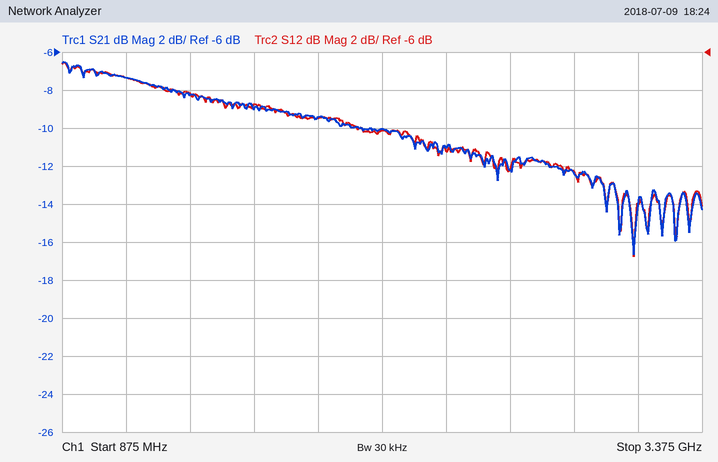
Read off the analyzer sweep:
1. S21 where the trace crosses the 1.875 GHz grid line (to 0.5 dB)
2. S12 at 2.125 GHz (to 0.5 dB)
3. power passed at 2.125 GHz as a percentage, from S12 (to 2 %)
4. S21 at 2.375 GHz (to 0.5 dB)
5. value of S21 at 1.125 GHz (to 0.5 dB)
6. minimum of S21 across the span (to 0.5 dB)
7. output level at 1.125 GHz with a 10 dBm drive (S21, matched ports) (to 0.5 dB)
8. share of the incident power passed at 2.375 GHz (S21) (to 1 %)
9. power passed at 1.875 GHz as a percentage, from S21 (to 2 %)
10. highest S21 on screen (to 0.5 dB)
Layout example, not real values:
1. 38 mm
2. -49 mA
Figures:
1. -9.5 dB
2. -10.0 dB
3. 10 %
4. -11.0 dB
5. -7.5 dB
6. -16.5 dB
7. 2.5 dBm
8. 8 %
9. 12 %
10. -6.5 dB
